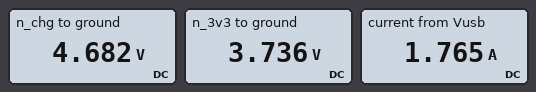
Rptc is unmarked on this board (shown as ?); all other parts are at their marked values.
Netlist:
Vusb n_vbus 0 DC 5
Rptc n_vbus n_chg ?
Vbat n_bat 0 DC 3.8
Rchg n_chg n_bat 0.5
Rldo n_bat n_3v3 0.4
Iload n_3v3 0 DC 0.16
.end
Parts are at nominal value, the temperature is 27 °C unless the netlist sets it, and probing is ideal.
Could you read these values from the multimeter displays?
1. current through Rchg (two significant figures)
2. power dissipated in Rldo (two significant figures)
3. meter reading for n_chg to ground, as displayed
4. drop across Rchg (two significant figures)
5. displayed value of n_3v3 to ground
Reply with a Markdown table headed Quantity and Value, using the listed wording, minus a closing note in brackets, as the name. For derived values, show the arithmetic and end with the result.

| Quantity | Value |
|---|---|
| current through Rchg | (4.682 V - 3.8 V) / 500 mΩ = 1.8 A |
| power dissipated in Rldo | (3.8 V - 3.736 V)^2 / 400 mΩ = 10 mW |
| meter reading for n_chg to ground, as displayed | 4.682 V |
| drop across Rchg | 4.682 V - 3.8 V = 880 mV |
| displayed value of n_3v3 to ground | 3.736 V |
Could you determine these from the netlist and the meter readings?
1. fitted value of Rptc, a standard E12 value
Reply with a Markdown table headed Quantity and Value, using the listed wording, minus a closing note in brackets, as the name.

| Quantity | Value |
|---|---|
| fitted value of Rptc, a standard E12 value | 0.18 Ω |
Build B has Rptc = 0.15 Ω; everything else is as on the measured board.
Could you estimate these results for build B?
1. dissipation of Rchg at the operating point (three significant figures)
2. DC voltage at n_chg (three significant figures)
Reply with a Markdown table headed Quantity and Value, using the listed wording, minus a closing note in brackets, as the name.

| Quantity | Value |
|---|---|
| dissipation of Rchg at the operating point | 1.70 W |
| DC voltage at n_chg | 4.72 V |
